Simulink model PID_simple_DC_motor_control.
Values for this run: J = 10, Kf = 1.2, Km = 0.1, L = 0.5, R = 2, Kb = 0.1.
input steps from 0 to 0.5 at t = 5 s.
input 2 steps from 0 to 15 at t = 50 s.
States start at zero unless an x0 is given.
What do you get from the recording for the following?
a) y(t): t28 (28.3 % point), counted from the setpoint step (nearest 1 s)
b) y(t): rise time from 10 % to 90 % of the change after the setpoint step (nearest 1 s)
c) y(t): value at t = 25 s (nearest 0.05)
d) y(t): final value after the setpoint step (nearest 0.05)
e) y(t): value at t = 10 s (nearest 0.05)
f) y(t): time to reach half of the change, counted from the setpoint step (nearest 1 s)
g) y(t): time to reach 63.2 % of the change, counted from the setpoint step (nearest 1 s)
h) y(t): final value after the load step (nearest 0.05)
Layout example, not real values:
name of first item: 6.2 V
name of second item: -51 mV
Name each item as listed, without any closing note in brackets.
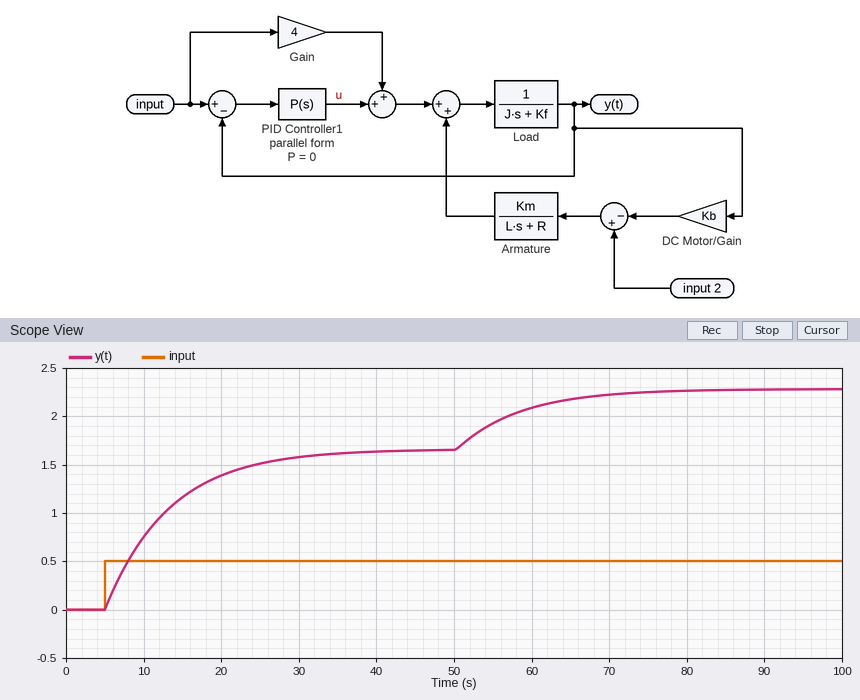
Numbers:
y(t): t28 (28.3 % point), counted from the setpoint step: 3 s
y(t): rise time from 10 % to 90 % of the change after the setpoint step: 18 s
y(t): value at t = 25 s: 1.50
y(t): final value after the setpoint step: 1.65
y(t): value at t = 10 s: 0.75
y(t): time to reach half of the change, counted from the setpoint step: 6 s
y(t): time to reach 63.2 % of the change, counted from the setpoint step: 8 s
y(t): final value after the load step: 2.30
